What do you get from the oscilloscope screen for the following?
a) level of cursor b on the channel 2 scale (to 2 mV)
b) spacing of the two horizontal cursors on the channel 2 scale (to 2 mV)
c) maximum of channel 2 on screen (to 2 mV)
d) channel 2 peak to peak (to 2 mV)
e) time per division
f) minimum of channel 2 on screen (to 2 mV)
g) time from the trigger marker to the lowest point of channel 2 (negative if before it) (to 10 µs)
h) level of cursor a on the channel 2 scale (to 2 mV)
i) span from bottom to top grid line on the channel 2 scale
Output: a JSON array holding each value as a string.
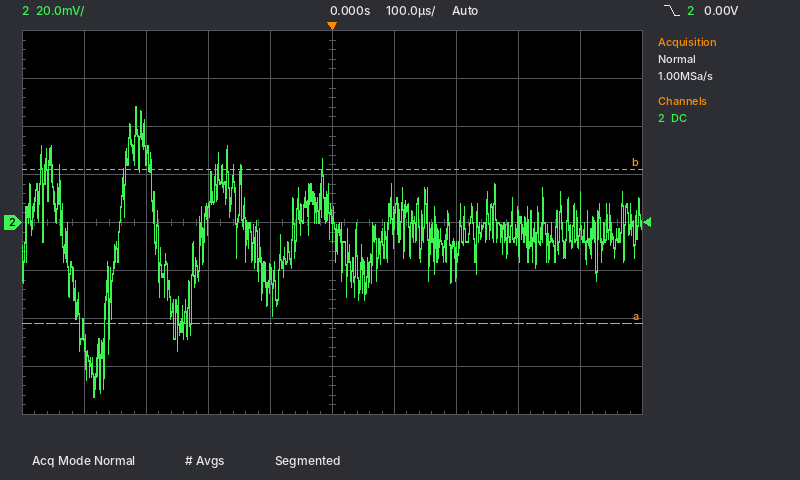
["22 mV", "64 mV", "48 mV", "120 mV", "100 µs", "-72 mV", "-380 µs", "-42 mV", "160 mV"]
